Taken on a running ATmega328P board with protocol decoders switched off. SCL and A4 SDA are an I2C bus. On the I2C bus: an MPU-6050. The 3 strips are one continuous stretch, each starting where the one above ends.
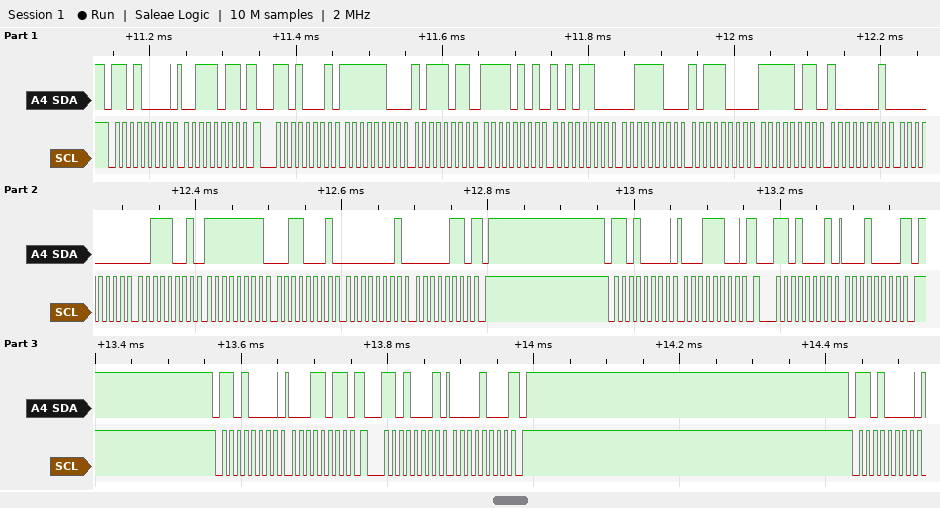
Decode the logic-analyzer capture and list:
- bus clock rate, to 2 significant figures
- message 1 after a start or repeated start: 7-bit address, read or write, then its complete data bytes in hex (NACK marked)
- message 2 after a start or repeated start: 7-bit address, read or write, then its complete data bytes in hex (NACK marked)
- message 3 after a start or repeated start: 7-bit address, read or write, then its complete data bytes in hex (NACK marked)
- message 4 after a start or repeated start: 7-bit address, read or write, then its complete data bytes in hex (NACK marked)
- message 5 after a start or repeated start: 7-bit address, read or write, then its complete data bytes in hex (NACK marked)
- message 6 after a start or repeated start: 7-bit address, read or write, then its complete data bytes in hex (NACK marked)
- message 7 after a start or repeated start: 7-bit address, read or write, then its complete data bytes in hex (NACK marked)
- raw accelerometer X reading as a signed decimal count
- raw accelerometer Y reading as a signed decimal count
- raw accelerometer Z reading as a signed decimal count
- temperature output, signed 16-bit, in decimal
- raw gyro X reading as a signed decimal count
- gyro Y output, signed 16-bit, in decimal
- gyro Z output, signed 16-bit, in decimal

100 kHz
0x68 write: 3B
0x68 read: FC BB F5 AC 3C B8 FB 81 00 39 FF 31 01 06 NACK
0x68 write: 1C
0x68 read: 10 NACK
0x68 write: 1B
0x68 read: 08 NACK
0x68 write
-837
-2644
15544
-1151
57
-207
262
